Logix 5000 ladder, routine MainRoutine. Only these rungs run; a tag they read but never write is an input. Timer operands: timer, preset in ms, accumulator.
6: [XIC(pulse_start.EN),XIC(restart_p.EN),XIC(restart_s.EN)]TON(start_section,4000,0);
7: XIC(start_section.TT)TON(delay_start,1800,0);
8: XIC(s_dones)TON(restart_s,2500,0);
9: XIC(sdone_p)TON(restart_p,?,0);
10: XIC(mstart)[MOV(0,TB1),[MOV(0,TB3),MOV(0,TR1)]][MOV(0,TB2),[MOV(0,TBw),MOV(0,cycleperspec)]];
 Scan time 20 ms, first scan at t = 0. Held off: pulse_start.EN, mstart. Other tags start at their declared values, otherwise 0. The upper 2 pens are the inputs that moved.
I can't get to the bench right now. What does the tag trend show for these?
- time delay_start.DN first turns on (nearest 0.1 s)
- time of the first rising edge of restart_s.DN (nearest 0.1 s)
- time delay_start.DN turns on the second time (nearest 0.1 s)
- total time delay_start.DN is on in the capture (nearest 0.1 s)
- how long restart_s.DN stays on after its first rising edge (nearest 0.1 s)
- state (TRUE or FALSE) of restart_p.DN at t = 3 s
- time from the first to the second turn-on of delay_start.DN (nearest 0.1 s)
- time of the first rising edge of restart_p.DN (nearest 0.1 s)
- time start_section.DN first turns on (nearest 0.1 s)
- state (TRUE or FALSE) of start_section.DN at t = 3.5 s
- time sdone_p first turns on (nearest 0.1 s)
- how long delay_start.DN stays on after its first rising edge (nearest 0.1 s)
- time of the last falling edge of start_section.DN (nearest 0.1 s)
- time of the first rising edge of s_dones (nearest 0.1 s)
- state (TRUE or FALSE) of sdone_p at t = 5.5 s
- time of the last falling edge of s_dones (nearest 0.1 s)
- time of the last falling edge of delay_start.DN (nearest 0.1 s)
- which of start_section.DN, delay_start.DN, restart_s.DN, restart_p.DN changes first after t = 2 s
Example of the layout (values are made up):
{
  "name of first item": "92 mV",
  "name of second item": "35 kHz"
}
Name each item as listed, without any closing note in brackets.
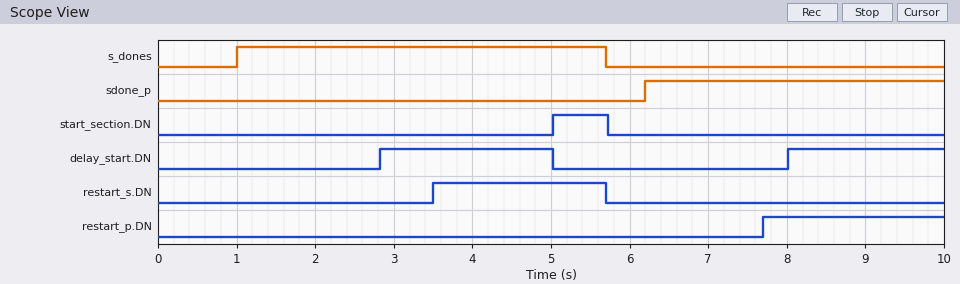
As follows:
{
  "time delay_start.DN first turns on": "2.8 s",
  "time of the first rising edge of restart_s.DN": "3.5 s",
  "time delay_start.DN turns on the second time": "8.0 s",
  "total time delay_start.DN is on in the capture": "4.2 s",
  "how long restart_s.DN stays on after its first rising edge": "2.2 s",
  "state (TRUE or FALSE) of restart_p.DN at t = 3 s": "FALSE",
  "time from the first to the second turn-on of delay_start.DN": "5.2 s",
  "time of the first rising edge of restart_p.DN": "7.7 s",
  "time start_section.DN first turns on": "5.0 s",
  "state (TRUE or FALSE) of start_section.DN at t = 3.5 s": "FALSE",
  "time sdone_p first turns on": "6.2 s",
  "how long delay_start.DN stays on after its first rising edge": "2.2 s",
  "time of the last falling edge of start_section.DN": "5.7 s",
  "time of the first rising edge of s_dones": "1.0 s",
  "state (TRUE or FALSE) of sdone_p at t = 5.5 s": "FALSE",
  "time of the last falling edge of s_dones": "5.7 s",
  "time of the last falling edge of delay_start.DN": "5.0 s",
  "which of start_section.DN, delay_start.DN, restart_s.DN, restart_p.DN changes first after t = 2 s": "delay_start.DN"
}
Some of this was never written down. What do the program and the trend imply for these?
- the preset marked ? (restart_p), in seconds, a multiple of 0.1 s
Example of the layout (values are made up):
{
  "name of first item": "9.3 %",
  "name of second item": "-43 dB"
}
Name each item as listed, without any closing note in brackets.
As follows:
{
  "the preset marked ? (restart_p), in seconds, a multiple of 0.1 s": "1.5 s"
}
